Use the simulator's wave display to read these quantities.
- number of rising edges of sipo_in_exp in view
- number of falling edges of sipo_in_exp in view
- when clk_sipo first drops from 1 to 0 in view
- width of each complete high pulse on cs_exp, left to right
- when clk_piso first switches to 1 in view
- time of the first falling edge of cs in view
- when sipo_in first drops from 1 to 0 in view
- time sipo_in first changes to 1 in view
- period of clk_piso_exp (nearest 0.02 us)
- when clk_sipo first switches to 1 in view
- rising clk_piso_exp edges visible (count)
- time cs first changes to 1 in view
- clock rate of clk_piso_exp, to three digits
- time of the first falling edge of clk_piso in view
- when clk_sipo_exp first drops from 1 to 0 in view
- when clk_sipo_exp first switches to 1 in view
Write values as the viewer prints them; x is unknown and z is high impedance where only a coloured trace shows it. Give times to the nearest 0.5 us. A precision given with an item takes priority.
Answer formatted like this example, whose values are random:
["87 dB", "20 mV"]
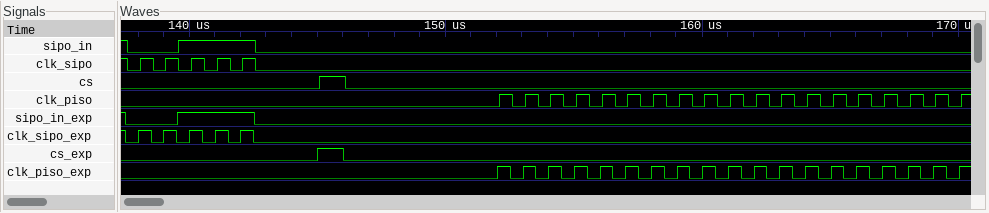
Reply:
["1", "2", "137.5 us", "1 us", "152 us", "146 us", "137.5 us", "139.5 us", "1 us", "138 us", "19", "145 us", "1.00 MHz", "152.5 us", "137.5 us", "138 us"]
